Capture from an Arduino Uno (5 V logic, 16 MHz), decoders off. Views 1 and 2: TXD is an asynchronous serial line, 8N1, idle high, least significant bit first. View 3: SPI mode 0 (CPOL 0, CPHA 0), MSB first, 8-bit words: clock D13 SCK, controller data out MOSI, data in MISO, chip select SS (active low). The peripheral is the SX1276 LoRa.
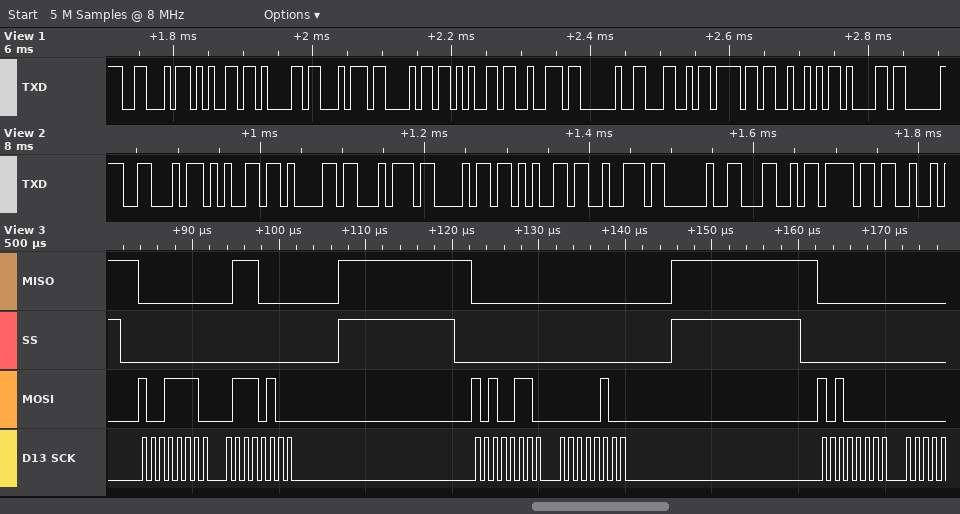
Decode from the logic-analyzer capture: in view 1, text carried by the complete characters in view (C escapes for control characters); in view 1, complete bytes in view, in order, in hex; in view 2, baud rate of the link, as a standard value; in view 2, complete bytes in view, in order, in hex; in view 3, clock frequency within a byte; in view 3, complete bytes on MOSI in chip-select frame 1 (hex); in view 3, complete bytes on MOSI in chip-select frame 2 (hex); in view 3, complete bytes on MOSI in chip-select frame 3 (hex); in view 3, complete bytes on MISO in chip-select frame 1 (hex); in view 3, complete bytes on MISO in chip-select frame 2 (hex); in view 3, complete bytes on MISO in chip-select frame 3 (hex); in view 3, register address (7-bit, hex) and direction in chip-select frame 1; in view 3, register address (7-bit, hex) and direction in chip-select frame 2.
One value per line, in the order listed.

"Feather LoRa"
0x46 0x65 0x61 0x74 0x68 0x65 0x72 0x20 0x4C 0x6F 0x52 0x61
115200 baud
0x46 0x65 0x61 0x74 0x68 0x65 0x72 0x20 0x4C 0x6F
1 MHz
0x9E 0x74
0xA6 0x04
0xA0
0x00 0x70
0x00 0x00
0x00
0x1E write
0x26 write
